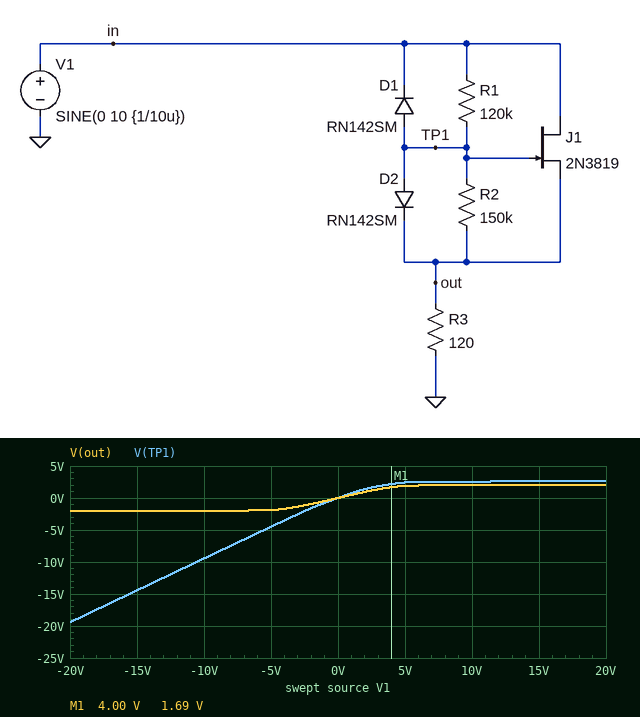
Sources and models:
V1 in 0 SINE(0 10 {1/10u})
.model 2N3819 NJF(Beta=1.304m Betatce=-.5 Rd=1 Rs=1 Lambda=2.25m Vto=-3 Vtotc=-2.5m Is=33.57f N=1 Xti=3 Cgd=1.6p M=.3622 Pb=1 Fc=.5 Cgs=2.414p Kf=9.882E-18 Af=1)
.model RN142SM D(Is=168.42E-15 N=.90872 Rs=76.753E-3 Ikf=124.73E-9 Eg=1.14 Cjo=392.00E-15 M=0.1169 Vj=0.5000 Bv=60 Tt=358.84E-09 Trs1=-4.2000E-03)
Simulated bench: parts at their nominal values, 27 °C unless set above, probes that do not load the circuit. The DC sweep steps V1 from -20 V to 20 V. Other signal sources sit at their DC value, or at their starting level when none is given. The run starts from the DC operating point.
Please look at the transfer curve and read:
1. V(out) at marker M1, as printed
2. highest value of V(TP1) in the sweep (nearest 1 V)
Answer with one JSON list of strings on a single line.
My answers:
["1.69 V", "3 V"]
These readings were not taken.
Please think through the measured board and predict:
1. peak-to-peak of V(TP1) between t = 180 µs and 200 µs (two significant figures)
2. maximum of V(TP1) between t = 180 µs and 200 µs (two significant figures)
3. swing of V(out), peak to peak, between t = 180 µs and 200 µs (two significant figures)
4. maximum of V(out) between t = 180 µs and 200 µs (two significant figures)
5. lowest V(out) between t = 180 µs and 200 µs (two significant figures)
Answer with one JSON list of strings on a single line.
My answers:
["12 V", "2.6 V", "4.0 V", "2.0 V", "-2.0 V"]
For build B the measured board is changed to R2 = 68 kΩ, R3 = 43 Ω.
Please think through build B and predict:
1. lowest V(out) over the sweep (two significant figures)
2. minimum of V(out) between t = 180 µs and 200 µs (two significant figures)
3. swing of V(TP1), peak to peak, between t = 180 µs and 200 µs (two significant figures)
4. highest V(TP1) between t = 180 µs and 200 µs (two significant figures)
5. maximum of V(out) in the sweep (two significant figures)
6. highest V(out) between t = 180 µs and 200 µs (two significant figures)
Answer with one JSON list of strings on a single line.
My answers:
["-760 mV", "-730 mV", "11 V", "1.3 V", "750 mV", "720 mV"]
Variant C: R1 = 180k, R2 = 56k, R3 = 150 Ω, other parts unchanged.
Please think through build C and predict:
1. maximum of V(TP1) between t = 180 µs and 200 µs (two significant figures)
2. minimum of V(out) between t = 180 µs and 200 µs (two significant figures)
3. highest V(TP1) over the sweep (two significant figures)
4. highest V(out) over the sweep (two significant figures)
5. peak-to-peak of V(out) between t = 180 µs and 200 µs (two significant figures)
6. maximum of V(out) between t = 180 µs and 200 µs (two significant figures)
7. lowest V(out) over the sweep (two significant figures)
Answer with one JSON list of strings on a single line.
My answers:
["3.0 V", "-2.5 V", "3.1 V", "2.6 V", "5.0 V", "2.5 V", "-2.7 V"]
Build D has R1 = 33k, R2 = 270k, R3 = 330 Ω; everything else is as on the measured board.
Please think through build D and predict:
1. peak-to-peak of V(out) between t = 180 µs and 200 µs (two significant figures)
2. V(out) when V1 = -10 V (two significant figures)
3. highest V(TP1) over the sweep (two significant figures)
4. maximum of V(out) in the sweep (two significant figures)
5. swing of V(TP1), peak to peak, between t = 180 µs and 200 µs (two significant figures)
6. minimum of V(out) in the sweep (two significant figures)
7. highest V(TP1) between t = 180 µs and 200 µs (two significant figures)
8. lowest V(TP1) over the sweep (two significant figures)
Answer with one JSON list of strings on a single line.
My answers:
["11 V", "-5.1 V", "6.5 V", "5.9 V", "16 V", "-5.5 V", "6.1 V", "-19 V"]
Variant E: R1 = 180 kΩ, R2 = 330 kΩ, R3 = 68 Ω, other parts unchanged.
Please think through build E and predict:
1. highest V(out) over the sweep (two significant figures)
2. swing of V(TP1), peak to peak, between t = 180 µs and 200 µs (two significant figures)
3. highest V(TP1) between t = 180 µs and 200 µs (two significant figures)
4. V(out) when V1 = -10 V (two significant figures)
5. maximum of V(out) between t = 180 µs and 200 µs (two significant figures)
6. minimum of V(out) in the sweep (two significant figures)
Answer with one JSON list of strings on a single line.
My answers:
["1.2 V", "11 V", "1.7 V", "-1.1 V", "1.1 V", "-1.2 V"]
